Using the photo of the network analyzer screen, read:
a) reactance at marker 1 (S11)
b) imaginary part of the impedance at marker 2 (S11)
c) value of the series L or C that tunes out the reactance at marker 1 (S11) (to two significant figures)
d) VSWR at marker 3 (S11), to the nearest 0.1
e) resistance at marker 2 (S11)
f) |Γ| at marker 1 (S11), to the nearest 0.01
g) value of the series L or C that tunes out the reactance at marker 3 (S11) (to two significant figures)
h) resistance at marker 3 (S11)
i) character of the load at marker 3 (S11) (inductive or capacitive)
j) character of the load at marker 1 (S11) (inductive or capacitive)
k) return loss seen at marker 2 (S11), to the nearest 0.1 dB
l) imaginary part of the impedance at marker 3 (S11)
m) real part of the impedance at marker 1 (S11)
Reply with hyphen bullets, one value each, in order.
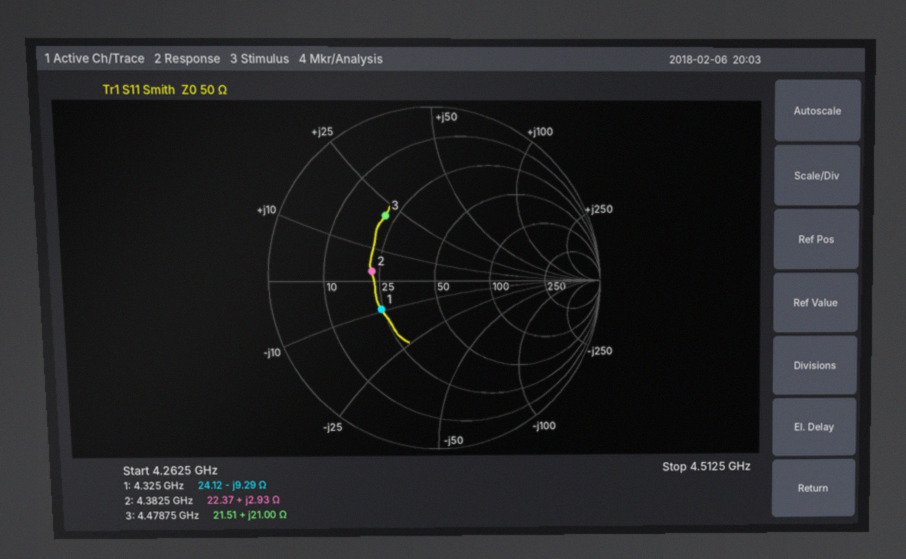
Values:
- -9.29 Ω
- +2.93 Ω
- 340 pH
- 2.8
- 22.37 Ω
- 0.37
- 1.7 pF
- 21.51 Ω
- inductive
- capacitive
- 8.3 dB
- +21.00 Ω
- 24.12 Ω
